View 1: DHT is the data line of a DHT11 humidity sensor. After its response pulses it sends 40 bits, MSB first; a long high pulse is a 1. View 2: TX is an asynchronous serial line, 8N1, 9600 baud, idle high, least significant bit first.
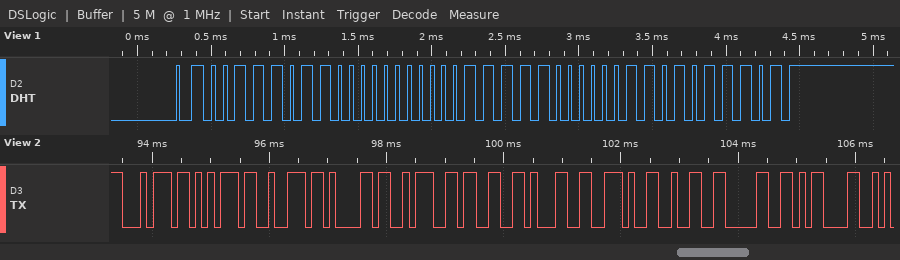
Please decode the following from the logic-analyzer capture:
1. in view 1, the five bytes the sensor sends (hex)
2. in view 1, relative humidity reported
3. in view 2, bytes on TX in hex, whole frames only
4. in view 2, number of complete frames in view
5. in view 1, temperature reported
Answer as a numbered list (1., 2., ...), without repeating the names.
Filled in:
1. 3B 00 1F 03 5D
2. 59 %
3. 74 75 72 61 3A 33 31 2E 32 30 0D
4. 11
5. 31.3 °C
